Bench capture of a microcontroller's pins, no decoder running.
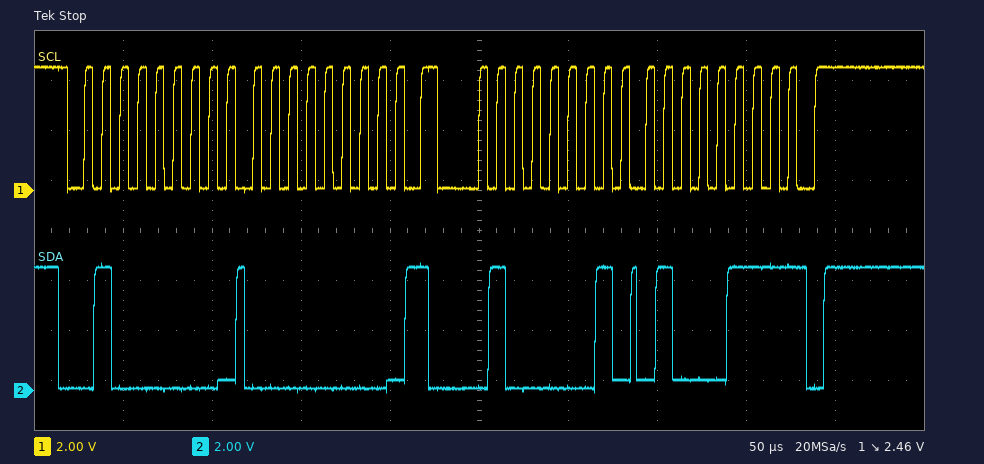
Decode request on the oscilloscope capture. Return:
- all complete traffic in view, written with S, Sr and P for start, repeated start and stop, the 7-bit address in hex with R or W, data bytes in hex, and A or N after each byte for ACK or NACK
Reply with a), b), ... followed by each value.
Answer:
a) S 20W A 00 A Sr 20R A 47 N P
